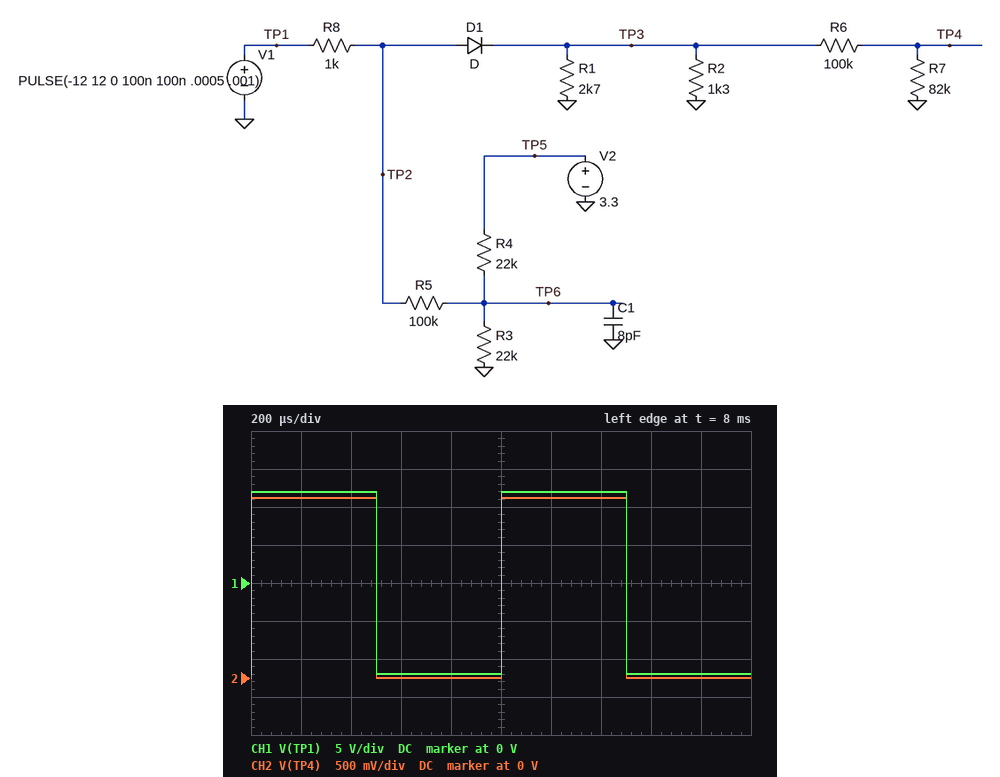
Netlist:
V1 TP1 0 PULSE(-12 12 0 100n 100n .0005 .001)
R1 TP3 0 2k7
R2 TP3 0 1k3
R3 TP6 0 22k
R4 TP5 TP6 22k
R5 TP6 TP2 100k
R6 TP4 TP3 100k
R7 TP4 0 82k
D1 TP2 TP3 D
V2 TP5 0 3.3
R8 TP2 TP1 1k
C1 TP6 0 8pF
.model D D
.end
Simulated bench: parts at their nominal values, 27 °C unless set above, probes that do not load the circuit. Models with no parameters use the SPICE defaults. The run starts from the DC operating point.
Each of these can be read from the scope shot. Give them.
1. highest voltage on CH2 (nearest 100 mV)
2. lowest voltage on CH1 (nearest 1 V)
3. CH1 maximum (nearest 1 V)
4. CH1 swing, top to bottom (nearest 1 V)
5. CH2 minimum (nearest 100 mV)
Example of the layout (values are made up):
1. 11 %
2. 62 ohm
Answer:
1. 2.4 V
2. -12 V
3. 12 V
4. 24 V
5. 0 V
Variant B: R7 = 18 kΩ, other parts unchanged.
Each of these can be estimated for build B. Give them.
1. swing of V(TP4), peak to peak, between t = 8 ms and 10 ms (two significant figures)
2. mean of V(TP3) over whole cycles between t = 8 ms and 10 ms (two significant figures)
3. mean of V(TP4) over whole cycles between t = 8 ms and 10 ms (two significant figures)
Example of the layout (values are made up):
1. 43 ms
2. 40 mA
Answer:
1. 800 mV
2. 2.6 V
3. 400 mV
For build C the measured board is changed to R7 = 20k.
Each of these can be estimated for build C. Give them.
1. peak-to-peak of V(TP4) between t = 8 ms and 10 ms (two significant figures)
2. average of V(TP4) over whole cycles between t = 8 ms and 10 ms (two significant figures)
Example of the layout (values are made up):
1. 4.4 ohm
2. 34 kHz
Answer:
1. 870 mV
2. 440 mV
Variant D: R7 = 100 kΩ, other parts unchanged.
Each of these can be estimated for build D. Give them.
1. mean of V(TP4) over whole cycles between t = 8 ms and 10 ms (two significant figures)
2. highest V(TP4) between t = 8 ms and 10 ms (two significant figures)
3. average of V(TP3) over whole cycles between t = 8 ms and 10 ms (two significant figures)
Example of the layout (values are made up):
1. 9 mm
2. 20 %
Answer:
1. 1.3 V
2. 2.6 V
3. 2.6 V
